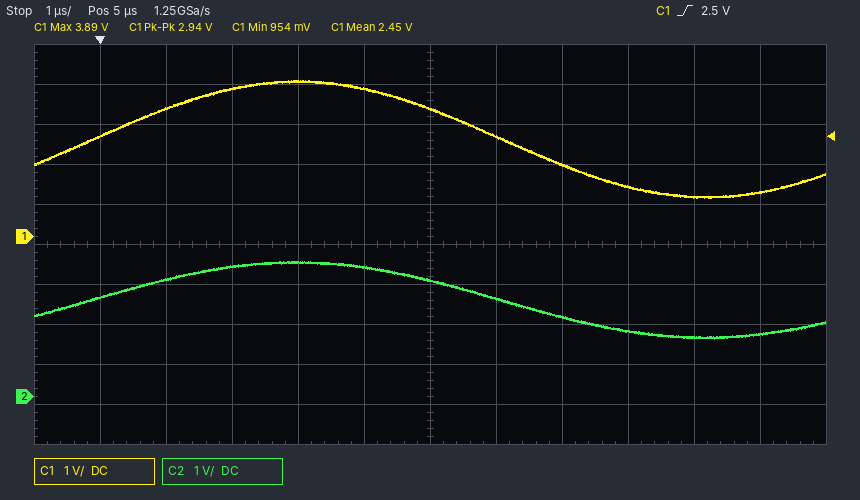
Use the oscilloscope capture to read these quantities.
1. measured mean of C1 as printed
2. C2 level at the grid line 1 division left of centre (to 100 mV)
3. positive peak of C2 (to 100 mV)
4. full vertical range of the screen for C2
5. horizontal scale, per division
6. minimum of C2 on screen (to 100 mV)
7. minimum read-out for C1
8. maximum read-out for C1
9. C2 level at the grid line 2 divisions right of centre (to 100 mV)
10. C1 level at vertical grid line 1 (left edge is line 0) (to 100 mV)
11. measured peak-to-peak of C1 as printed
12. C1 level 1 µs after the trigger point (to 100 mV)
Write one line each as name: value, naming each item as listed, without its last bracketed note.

measured mean of C1 as printed: 2.45 V
C2 level at the grid line 1 division left of centre: 3.2 V
positive peak of C2: 3.4 V
full vertical range of the screen for C2: 10 V
horizontal scale, per division: 1 µs
minimum of C2 on screen: 1.4 V
minimum read-out for C1: 954 mV
maximum read-out for C1: 3.89 V
C2 level at the grid line 2 divisions right of centre: 2.0 V
C1 level at vertical grid line 1 (left edge is line 0): 2.5 V
measured peak-to-peak of C1 as printed: 2.94 V
C1 level 1 µs after the trigger point: 3.2 V
